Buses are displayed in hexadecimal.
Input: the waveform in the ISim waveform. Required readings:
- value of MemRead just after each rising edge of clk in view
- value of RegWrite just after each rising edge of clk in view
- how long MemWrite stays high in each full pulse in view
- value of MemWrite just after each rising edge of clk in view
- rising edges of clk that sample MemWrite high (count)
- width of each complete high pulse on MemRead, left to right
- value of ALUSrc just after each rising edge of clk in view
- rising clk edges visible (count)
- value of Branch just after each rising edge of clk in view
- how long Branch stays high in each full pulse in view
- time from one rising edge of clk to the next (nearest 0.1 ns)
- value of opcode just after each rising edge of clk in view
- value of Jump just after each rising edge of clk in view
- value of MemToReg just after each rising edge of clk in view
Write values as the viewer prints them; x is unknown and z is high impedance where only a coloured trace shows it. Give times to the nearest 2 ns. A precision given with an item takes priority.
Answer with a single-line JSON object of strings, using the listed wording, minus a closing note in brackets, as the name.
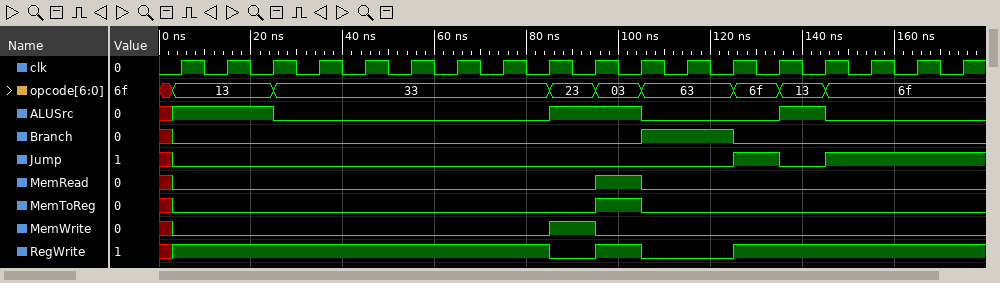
{"value of MemRead just after each rising edge of clk in view": "0 0 0 0 0 0 0 0 0 1 0 0 0 0 0 0 0 0", "value of RegWrite just after each rising edge of clk in view": "1 1 1 1 1 1 1 1 0 1 0 0 1 1 1 1 1 1", "how long MemWrite stays high in each full pulse in view": "10 ns", "value of MemWrite just after each rising edge of clk in view": "0 0 0 0 0 0 0 0 1 0 0 0 0 0 0 0 0 0", "rising edges of clk that sample MemWrite high": "1", "width of each complete high pulse on MemRead, left to right": "10 ns", "value of ALUSrc just after each rising edge of clk in view": "1 1 0 0 0 0 0 0 1 1 0 0 0 1 0 0 0 0", "rising clk edges visible": "18", "value of Branch just after each rising edge of clk in view": "0 0 0 0 0 0 0 0 0 0 1 1 0 0 0 0 0 0", "how long Branch stays high in each full pulse in view": "20 ns", "time from one rising edge of clk to the next": "10 ns", "value of opcode just after each rising edge of clk in view": "13, 13, 33, 33, 33, 33, 33, 33, 23, 03, 63, 63, 6f, 13, 6f, 6f, 6f, 6f", "value of Jump just after each rising edge of clk in view": "0 0 0 0 0 0 0 0 0 0 0 0 1 0 1 1 1 1", "value of MemToReg just after each rising edge of clk in view": "0 0 0 0 0 0 0 0 0 1 0 0 0 0 0 0 0 0"}
